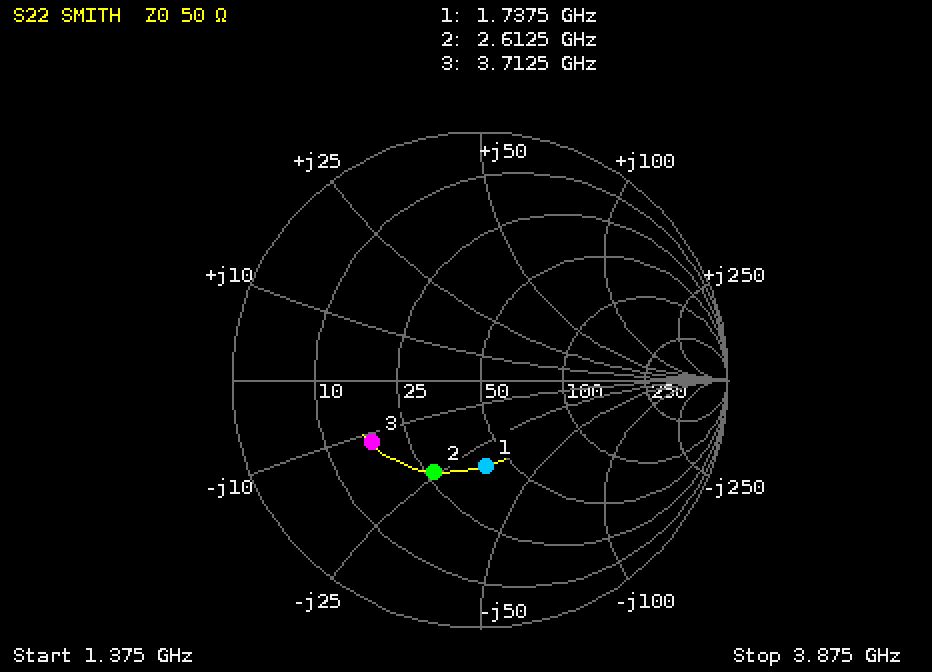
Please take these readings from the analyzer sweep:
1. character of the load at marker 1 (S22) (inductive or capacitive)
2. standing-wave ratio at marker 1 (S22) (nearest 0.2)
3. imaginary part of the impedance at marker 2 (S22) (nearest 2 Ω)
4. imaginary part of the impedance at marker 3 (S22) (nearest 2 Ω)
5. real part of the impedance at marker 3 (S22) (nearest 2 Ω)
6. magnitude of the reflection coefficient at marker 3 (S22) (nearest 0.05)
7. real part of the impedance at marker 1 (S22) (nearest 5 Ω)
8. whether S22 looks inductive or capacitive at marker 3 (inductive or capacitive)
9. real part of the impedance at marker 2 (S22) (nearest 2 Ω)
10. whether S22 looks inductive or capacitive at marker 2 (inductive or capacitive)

capacitive
2.0
-24 Ω
-12 Ω
18 Ω
0.50
40 Ω
capacitive
26 Ω
capacitive
